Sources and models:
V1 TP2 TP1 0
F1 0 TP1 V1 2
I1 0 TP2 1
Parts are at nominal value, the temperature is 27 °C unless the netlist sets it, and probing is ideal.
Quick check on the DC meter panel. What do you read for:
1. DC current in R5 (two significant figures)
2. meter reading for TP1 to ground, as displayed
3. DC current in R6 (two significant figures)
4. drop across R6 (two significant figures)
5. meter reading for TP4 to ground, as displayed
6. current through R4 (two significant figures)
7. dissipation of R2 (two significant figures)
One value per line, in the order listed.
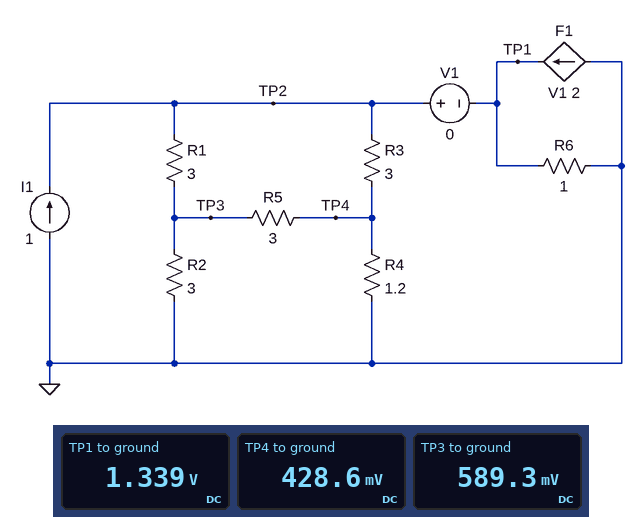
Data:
54 mA
1.339 V
1.3 A
1.3 V
428.6 mV
360 mA
120 mW
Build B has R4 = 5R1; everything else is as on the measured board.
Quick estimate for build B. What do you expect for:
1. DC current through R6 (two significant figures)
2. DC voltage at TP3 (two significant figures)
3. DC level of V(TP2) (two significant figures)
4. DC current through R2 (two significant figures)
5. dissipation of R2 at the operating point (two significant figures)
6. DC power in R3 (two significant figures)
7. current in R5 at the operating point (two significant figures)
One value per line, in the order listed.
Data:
1.6 A
850 mV
1.6 V
280 mA
240 mW
140 mW
32 mA
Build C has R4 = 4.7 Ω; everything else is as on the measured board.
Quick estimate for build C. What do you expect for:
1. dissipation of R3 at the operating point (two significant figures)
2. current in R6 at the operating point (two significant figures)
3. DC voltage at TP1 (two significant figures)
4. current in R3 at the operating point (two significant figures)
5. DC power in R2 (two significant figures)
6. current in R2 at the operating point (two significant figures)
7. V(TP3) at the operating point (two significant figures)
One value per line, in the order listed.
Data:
150 mW
1.6 A
1.6 V
220 mA
230 mW
280 mA
830 mV
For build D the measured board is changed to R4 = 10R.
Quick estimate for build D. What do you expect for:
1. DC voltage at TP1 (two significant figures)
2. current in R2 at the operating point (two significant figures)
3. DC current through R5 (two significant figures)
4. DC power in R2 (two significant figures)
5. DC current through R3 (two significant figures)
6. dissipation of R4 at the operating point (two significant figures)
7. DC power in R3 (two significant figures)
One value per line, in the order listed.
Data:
1.7 V
320 mA
67 mA
300 mW
180 mA
130 mW
100 mW
